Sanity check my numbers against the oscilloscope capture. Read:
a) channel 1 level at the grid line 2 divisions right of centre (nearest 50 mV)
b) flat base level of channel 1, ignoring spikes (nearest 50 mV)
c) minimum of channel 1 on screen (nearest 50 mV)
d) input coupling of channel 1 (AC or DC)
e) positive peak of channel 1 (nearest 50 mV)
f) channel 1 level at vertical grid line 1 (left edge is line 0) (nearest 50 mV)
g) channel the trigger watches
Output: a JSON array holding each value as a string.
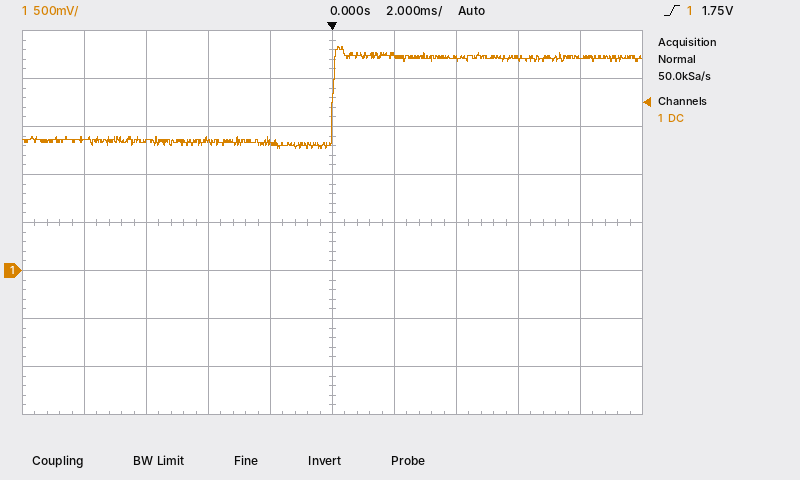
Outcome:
["2.20 V", "1.35 V", "1.25 V", "DC", "2.35 V", "1.35 V", "channel 1"]
